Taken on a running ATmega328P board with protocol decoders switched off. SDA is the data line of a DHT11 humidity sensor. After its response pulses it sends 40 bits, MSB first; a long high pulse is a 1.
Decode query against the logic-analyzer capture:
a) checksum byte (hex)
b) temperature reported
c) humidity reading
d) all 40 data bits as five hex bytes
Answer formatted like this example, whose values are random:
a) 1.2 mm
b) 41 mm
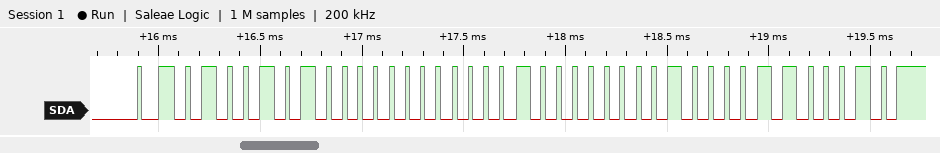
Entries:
a) 0x62
b) 16.8 °C
c) 74 %
d) 4A 00 10 08 62
